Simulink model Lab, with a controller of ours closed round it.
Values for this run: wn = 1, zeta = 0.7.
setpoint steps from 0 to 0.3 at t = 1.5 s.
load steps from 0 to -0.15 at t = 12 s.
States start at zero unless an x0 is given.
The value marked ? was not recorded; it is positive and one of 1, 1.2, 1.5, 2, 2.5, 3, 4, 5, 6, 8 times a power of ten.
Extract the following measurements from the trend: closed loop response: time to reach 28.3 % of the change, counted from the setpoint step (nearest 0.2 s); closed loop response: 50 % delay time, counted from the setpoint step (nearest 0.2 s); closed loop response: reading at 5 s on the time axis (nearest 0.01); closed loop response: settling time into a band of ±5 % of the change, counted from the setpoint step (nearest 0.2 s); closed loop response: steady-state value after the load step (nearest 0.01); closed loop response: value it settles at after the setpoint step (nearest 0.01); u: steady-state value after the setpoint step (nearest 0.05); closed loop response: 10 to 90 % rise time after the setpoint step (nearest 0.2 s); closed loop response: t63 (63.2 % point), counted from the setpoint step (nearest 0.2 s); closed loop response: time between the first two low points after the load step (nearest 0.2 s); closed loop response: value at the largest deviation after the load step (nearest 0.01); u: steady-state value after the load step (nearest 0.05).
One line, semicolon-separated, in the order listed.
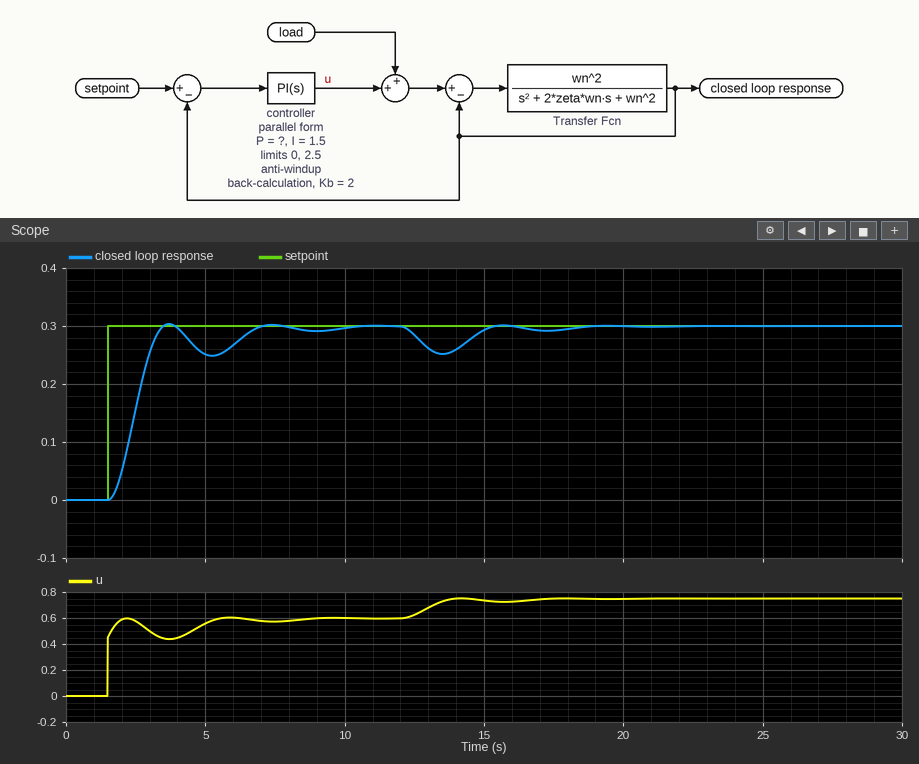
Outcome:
0.6 s; 1.0 s; 0.25; 5.0 s; 0.30; 0.30; 0.60; 1.2 s; 1.2 s; 3.8 s; 0.25; 0.75
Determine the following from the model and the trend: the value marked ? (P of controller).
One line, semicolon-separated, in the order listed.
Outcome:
1.5
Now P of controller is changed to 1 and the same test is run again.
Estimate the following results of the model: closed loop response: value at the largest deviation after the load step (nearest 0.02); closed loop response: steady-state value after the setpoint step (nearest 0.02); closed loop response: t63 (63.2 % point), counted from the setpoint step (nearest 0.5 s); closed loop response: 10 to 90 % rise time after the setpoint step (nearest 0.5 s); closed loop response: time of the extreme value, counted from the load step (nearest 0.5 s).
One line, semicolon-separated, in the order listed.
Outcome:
0.24; 0.30; 1.5 s; 1.5 s; 1.5 s
